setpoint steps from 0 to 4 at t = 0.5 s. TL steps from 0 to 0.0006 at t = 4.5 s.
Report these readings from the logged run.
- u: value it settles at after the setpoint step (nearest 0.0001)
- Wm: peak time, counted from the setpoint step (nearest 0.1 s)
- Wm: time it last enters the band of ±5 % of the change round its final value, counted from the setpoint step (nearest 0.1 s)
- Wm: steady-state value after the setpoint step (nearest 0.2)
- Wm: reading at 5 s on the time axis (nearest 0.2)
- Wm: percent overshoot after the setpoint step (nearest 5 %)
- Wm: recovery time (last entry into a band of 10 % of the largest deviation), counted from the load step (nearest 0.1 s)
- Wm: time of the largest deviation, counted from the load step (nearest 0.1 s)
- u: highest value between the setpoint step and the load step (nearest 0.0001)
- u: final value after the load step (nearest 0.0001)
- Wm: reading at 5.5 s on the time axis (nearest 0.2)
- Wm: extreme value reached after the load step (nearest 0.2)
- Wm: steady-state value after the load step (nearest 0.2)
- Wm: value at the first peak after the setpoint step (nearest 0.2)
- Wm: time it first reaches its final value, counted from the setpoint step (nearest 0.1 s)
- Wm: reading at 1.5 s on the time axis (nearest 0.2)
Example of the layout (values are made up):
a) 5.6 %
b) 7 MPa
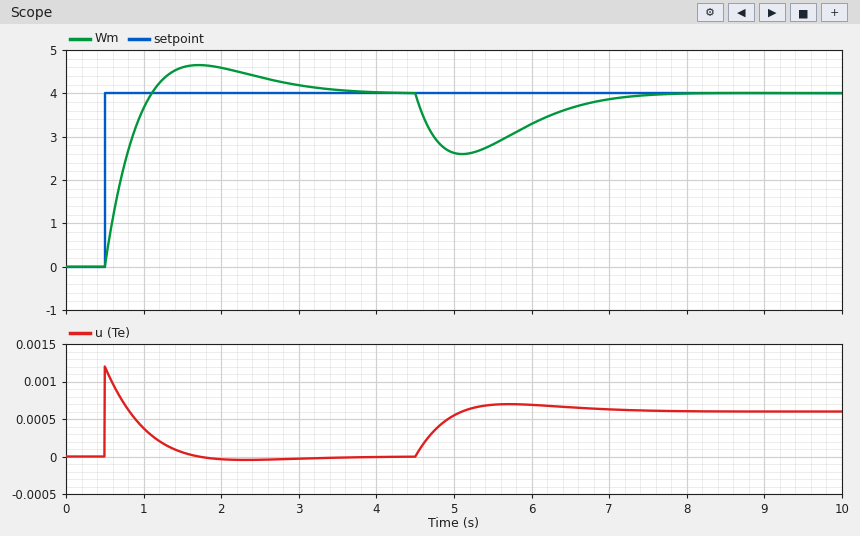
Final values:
a) 0.0000
b) 1.2 s
c) 2.5 s
d) 4.0
e) 2.6
f) 15 %
g) 2.5 s
h) 0.6 s
i) 0.0012
j) 0.0006
k) 2.8
l) 2.6
m) 4.0
n) 4.6
o) 0.6 s
p) 4.6
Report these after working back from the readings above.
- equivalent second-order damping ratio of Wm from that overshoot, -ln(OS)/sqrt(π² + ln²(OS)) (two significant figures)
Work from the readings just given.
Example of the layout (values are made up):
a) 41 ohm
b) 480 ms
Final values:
a) 0.52
